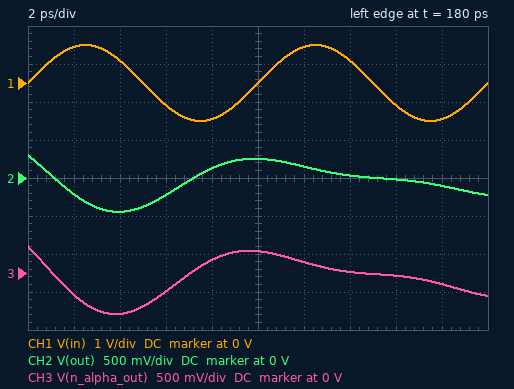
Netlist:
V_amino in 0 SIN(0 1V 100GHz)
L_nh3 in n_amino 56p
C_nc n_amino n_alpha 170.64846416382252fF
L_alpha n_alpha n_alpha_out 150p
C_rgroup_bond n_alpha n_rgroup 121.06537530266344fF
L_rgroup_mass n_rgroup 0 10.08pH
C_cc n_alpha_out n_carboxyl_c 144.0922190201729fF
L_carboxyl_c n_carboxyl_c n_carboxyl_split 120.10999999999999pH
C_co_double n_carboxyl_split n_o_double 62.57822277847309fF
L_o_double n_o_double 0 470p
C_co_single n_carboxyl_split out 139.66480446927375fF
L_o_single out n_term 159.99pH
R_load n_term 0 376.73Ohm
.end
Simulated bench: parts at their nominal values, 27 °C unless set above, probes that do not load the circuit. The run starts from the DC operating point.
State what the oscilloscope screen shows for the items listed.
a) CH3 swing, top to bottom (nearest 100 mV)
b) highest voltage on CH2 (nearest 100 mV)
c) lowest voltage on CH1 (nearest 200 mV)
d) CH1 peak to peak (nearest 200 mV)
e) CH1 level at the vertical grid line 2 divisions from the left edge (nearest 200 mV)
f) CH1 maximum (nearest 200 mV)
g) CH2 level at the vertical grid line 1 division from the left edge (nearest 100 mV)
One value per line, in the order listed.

900 mV
300 mV
-1.0 V
2.0 V
600 mV
1.0 V
-200 mV
